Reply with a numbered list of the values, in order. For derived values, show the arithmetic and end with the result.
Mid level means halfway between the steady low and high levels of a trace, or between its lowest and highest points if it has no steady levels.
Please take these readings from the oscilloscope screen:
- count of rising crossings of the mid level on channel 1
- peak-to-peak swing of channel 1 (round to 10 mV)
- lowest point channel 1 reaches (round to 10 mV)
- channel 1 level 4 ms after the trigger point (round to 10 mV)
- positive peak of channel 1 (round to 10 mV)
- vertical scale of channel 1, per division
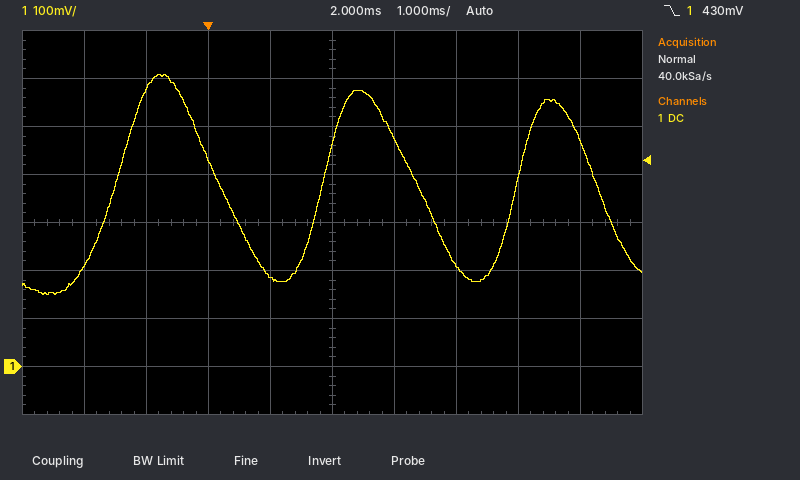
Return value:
1. 3
2. 610 mV − (150 mV) = 460 mV
3. 150 mV
4. 210 mV
5. 610 mV
6. 100 mV
